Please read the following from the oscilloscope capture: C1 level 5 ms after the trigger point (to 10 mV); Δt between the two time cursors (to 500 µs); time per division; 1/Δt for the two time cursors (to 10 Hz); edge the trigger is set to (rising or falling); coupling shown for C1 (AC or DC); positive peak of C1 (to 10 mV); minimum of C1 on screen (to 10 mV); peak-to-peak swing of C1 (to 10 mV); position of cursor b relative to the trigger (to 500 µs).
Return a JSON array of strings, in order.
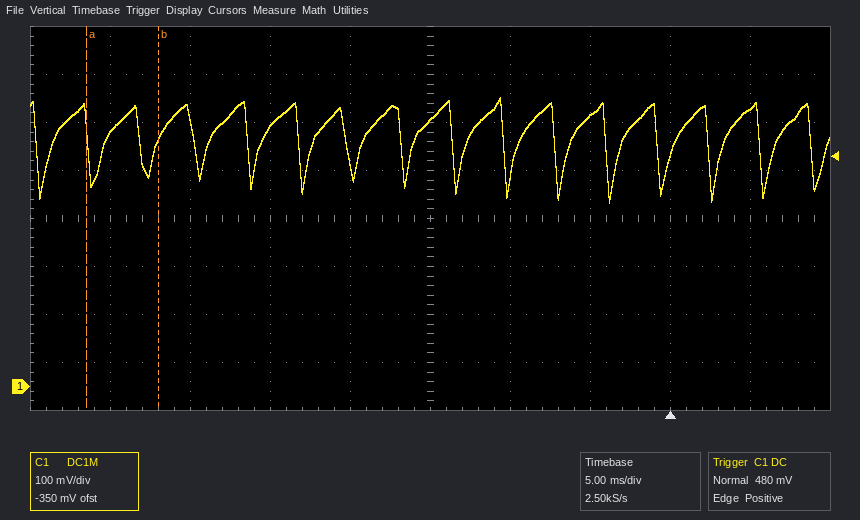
["580 mV", "4.5 ms", "5 ms", "220 Hz", "rising", "DC", "600 mV", "380 mV", "220 mV", "-32.0 ms"]
